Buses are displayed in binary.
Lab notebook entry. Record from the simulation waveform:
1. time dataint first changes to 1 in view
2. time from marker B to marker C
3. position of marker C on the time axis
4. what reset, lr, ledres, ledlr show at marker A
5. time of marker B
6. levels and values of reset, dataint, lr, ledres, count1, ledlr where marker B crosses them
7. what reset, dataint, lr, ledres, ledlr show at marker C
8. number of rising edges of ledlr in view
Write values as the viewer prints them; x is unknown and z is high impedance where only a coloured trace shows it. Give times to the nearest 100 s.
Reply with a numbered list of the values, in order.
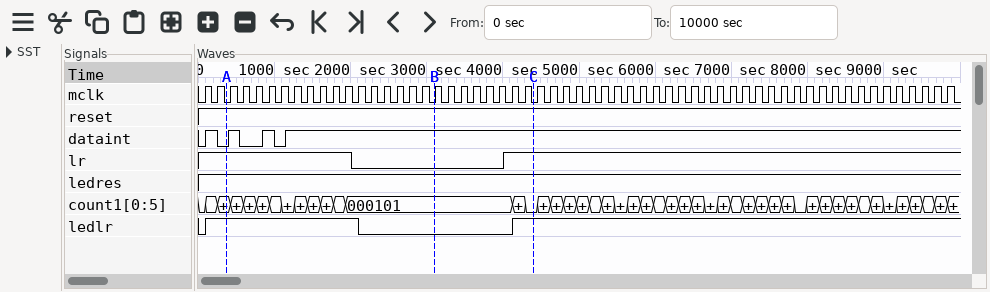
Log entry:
1. 100 s
2. 1300 s
3. 4400 s
4. reset=1, lr=1, ledres=1, ledlr=1
5. 3100 s
6. reset=1, dataint=1, lr=0, ledres=1, count1=000101, ledlr=0
7. reset=1, dataint=1, lr=1, ledres=1, ledlr=1
8. 2
